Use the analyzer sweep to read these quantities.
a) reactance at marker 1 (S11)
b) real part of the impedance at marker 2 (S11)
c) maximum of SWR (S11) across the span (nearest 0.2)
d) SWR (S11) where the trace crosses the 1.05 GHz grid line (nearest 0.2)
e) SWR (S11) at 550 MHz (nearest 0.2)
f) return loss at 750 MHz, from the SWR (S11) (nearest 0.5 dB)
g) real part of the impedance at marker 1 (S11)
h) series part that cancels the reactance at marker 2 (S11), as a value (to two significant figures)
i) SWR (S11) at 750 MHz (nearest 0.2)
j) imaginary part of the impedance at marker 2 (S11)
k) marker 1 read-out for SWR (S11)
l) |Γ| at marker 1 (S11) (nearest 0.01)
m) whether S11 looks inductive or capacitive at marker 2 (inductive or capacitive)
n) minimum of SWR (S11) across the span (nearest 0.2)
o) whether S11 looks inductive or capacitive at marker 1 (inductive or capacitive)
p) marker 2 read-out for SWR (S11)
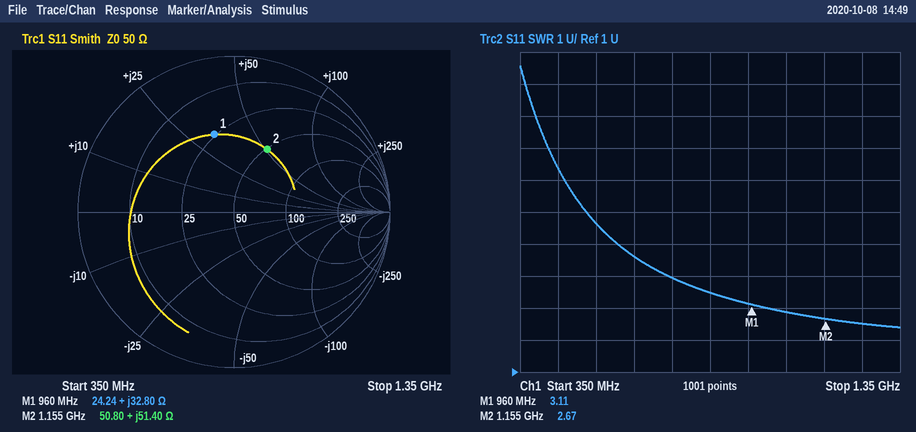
+32.80 Ω
50.80 Ω
10.6
2.8
5.6
4.5 dB
24.24 Ω
2.7 pF
4.0
+51.40 Ω
3.11
0.51
inductive
2.4
inductive
2.67
